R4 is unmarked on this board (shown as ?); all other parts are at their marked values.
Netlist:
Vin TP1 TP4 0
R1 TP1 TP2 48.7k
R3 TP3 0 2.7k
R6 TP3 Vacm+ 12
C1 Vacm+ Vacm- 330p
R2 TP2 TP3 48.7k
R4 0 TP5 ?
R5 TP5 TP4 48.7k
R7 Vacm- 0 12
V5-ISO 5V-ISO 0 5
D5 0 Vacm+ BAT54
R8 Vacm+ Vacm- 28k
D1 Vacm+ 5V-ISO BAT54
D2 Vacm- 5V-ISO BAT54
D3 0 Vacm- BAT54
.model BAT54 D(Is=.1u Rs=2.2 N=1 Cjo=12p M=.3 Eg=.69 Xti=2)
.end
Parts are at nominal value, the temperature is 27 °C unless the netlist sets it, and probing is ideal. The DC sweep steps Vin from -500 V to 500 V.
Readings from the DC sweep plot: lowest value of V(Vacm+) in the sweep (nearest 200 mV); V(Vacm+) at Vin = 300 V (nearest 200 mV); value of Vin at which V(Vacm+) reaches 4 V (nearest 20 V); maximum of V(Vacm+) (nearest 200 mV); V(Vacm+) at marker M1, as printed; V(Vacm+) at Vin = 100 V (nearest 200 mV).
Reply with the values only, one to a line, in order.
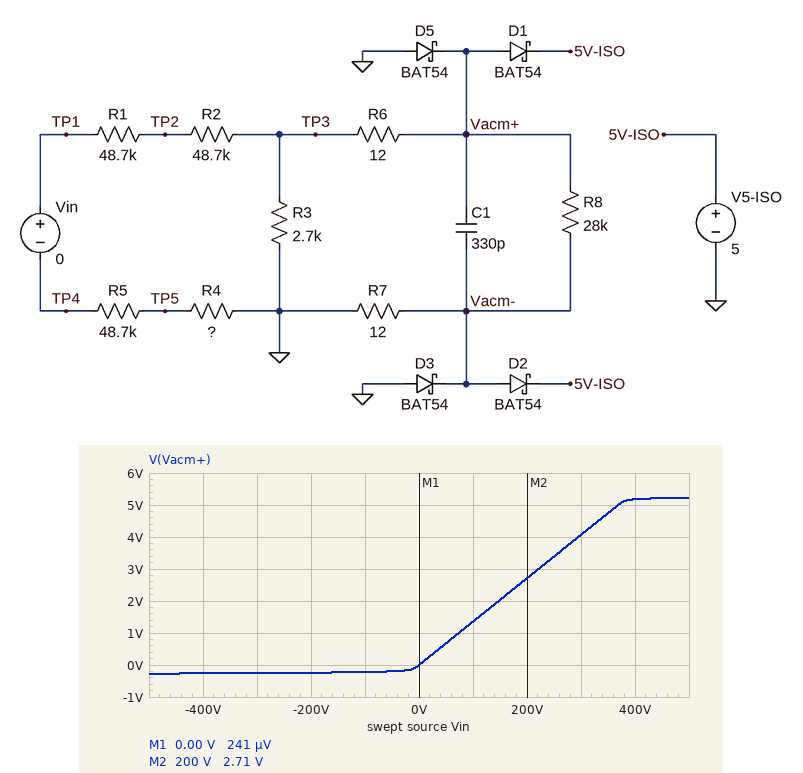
-200 mV
4.0 V
300 V
5.2 V
241 µV
1.4 V
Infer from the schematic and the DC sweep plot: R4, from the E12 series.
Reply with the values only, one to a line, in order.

33 kΩ
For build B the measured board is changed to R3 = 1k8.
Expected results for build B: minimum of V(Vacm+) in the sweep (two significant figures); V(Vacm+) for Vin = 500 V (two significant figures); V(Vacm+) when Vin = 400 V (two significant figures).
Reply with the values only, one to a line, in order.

-270 mV
4.7 V
3.7 V
